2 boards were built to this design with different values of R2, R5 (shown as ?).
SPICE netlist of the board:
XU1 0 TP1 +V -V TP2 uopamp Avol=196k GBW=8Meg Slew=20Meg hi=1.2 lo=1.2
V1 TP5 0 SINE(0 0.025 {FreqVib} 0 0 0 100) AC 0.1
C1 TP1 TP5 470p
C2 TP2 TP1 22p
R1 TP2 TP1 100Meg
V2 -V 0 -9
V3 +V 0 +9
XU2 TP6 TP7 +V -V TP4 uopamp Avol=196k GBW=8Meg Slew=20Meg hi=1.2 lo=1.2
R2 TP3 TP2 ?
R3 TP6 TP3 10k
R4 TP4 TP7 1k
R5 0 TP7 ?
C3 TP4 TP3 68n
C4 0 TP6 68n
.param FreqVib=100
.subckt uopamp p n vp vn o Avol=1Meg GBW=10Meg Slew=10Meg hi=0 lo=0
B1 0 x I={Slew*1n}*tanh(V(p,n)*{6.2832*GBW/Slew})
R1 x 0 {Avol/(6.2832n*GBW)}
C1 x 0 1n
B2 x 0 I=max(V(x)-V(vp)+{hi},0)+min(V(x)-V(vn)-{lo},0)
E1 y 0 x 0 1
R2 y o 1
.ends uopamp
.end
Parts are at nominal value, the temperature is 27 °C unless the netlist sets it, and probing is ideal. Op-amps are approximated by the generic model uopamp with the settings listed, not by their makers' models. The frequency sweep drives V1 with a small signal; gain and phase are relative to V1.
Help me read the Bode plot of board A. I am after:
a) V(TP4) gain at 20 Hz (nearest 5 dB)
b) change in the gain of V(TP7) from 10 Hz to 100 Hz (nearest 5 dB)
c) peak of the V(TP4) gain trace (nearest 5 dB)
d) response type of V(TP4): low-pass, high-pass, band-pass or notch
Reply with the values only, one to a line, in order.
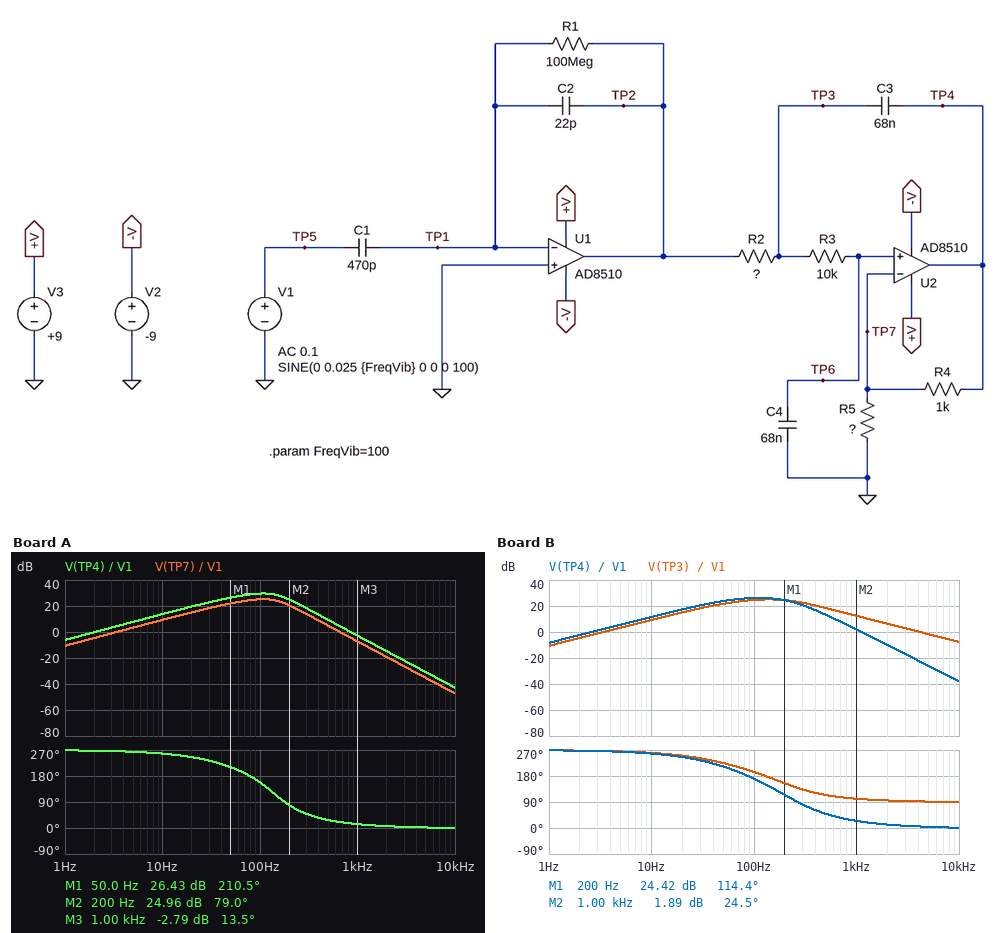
20 dB
15 dB
30 dB
band-pass
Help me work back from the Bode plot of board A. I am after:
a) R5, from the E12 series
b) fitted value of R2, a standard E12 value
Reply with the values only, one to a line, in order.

1.5 kΩ
27 kΩ
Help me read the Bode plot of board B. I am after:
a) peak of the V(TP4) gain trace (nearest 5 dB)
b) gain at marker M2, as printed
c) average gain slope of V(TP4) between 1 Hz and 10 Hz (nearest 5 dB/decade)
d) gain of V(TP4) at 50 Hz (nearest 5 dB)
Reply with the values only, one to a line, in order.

25 dB
1.89 dB
20 dB/decade
25 dB
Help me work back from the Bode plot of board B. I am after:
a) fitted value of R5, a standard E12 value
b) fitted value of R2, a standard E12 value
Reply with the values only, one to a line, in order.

3.3 kΩ
12 kΩ
